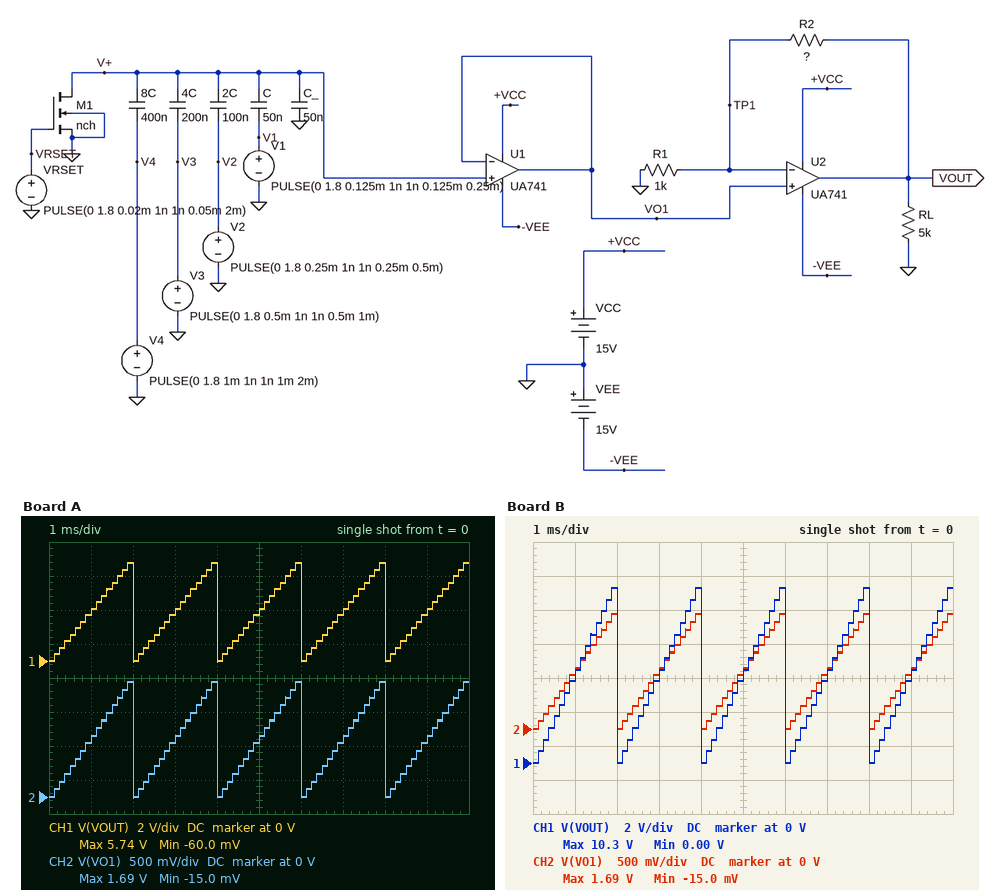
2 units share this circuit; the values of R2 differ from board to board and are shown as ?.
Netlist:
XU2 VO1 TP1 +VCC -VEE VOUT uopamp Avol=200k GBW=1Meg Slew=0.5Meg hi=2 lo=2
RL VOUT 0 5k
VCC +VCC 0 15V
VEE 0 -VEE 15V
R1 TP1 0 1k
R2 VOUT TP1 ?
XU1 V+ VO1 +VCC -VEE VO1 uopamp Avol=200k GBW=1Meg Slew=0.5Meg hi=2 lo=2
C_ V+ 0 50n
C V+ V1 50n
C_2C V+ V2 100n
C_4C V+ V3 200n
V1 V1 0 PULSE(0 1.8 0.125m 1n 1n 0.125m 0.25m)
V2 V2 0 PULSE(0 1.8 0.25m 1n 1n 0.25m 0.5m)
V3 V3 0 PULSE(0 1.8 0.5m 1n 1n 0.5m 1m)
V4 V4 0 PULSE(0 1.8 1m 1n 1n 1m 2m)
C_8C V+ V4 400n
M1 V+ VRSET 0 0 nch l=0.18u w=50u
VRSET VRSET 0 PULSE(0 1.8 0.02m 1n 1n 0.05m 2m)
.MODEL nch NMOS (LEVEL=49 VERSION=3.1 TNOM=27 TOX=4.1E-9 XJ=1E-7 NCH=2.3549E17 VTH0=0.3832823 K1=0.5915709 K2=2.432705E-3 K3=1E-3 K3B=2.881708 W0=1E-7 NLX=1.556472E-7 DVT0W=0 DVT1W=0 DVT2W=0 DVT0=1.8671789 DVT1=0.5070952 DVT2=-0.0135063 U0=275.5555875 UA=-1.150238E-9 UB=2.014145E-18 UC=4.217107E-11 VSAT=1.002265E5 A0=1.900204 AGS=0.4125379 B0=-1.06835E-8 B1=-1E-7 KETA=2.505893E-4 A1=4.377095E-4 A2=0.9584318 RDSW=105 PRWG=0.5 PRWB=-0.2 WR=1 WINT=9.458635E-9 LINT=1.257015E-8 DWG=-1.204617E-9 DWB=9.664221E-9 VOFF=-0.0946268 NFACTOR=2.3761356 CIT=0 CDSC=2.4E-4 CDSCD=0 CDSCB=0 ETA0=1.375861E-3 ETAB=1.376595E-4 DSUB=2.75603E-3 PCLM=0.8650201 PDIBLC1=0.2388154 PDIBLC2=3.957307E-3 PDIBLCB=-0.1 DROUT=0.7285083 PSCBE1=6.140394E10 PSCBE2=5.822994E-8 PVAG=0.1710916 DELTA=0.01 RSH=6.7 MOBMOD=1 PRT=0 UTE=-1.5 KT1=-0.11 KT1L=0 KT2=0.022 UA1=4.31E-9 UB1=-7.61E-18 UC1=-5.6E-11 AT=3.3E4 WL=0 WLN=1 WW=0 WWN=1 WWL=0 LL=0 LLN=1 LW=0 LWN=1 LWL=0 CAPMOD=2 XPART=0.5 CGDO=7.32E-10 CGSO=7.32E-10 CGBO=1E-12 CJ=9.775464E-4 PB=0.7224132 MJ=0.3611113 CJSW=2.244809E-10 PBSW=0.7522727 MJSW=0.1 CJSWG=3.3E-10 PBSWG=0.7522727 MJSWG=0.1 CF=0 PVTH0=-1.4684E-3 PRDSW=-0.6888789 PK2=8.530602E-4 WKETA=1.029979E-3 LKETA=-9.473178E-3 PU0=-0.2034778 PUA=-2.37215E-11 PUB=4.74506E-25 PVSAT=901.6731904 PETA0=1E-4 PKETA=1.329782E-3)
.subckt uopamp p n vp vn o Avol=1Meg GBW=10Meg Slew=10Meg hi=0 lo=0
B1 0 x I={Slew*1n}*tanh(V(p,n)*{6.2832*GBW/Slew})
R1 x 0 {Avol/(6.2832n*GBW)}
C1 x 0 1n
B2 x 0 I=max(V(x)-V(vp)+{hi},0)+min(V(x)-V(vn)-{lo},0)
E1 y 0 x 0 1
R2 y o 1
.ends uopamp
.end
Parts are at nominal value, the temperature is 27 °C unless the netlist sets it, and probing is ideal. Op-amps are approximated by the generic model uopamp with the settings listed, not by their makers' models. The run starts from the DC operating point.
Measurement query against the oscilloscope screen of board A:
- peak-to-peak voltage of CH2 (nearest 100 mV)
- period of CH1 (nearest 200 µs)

1.7 V
2.0 ms
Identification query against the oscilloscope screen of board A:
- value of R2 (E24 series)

2.4 kΩ
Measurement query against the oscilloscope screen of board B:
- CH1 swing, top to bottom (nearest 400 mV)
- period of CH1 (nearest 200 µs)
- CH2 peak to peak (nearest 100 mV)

10.4 V
2.0 ms
1.7 V
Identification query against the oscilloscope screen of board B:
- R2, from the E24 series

5.1 kΩ
